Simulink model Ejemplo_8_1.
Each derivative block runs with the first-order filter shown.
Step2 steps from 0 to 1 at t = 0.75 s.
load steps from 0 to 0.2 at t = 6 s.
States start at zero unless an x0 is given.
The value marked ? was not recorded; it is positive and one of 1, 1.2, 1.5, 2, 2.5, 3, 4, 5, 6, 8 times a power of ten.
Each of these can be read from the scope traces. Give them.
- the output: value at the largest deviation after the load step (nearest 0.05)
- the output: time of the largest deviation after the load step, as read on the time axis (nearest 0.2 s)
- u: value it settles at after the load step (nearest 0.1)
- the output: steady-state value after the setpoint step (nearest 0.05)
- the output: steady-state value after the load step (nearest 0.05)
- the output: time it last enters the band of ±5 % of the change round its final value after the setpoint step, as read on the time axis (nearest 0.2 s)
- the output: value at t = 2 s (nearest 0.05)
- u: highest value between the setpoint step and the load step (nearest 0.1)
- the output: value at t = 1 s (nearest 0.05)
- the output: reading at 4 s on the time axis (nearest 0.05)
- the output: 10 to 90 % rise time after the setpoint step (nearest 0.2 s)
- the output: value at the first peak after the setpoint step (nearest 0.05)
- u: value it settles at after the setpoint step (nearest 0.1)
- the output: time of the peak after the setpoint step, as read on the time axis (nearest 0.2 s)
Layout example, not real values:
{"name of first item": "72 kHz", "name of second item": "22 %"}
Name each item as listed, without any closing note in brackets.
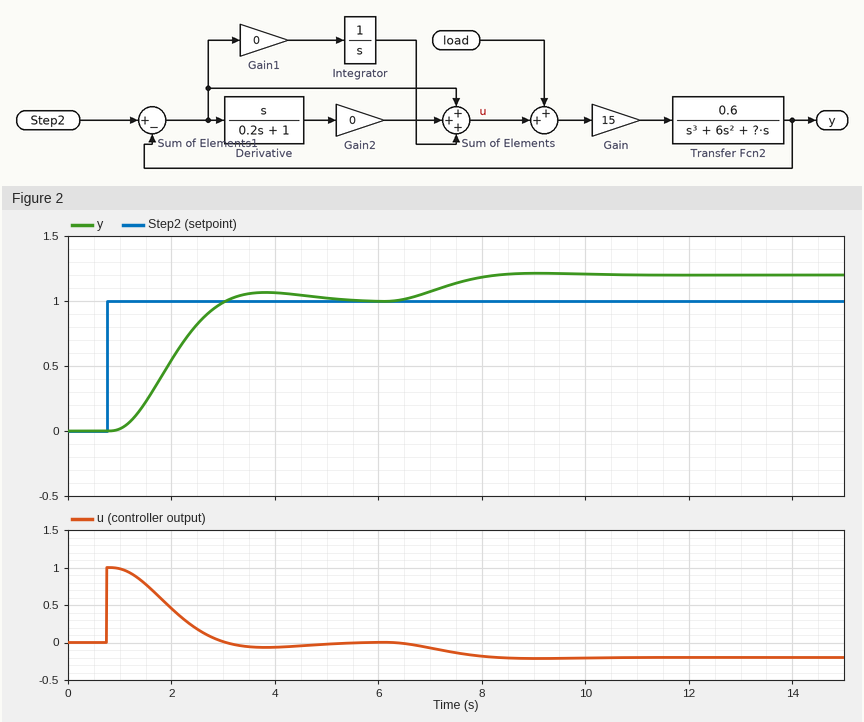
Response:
{"the output: value at the largest deviation after the load step": "1.20", "the output: time of the largest deviation after the load step, as read on the time axis": "9.0 s", "u: value it settles at after the load step": "-0.2", "the output: steady-state value after the setpoint step": "1.00", "the output: steady-state value after the load step": "1.20", "the output: time it last enters the band of ±5 % of the change round its final value after the setpoint step, as read on the time axis": "4.4 s", "the output: value at t = 2 s": "0.55", "u: highest value between the setpoint step and the load step": "1.0", "the output: value at t = 1 s": "0.00", "the output: reading at 4 s on the time axis": "1.05", "the output: 10 to 90 % rise time after the setpoint step": "1.4 s", "the output: value at the first peak after the setpoint step": "1.05", "u: value it settles at after the setpoint step": "0.0", "the output: time of the peak after the setpoint step, as read on the time axis": "3.8 s"}
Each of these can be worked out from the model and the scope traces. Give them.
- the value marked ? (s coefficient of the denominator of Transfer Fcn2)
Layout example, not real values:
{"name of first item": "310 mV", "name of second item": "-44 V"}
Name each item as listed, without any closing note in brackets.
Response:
{"the value marked ?": "10"}
